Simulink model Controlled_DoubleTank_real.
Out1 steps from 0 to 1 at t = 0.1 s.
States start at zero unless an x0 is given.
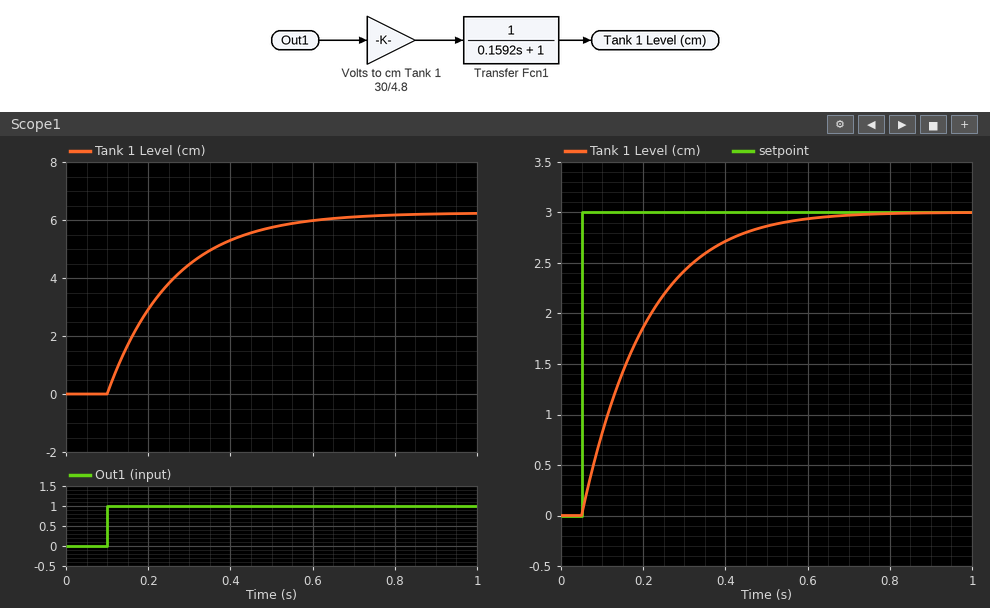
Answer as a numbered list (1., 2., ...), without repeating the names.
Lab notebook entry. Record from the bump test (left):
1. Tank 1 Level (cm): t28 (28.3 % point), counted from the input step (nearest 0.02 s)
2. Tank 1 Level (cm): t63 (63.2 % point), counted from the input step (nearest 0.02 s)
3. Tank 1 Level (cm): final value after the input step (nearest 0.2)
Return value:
1. 0.06 s
2. 0.16 s
3. 6.2
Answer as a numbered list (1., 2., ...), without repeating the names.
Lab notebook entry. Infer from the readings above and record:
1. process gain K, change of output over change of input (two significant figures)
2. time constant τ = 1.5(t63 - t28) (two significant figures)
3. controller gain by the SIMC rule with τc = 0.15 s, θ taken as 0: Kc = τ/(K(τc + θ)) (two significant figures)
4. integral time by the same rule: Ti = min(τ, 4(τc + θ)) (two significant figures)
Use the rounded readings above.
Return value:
1. 6.2
2. 0.15 s
3. 0.16
4. 0.15 s
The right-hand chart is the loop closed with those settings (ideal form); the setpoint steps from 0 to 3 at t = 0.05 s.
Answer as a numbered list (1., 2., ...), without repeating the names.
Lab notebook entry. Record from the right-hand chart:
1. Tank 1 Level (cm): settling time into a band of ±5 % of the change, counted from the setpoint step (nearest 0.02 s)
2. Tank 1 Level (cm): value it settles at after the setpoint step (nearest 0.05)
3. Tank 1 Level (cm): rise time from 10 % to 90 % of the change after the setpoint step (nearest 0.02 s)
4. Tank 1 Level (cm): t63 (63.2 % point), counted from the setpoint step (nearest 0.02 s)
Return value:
1. 0.44 s
2. 3.00
3. 0.32 s
4. 0.16 s
